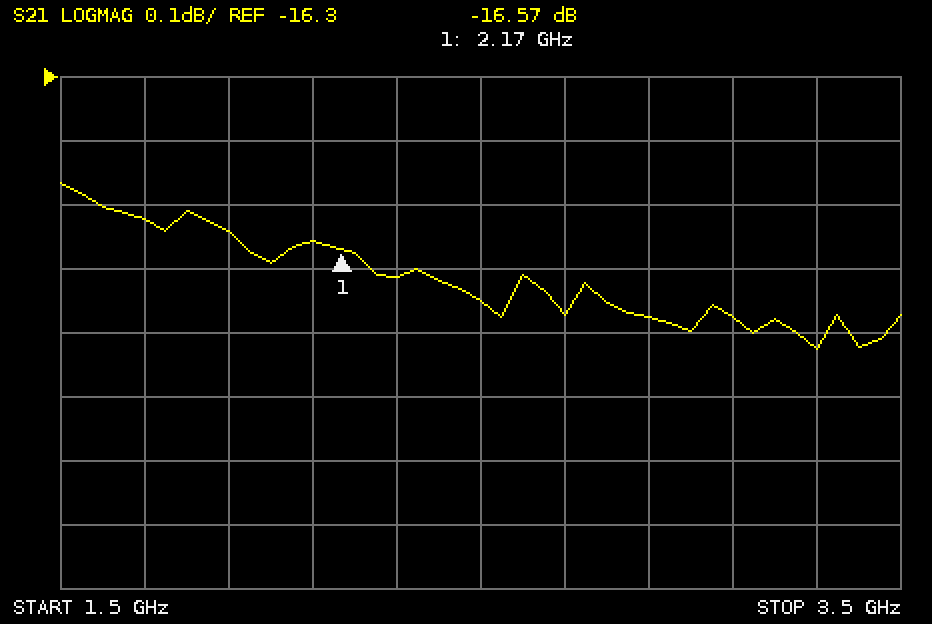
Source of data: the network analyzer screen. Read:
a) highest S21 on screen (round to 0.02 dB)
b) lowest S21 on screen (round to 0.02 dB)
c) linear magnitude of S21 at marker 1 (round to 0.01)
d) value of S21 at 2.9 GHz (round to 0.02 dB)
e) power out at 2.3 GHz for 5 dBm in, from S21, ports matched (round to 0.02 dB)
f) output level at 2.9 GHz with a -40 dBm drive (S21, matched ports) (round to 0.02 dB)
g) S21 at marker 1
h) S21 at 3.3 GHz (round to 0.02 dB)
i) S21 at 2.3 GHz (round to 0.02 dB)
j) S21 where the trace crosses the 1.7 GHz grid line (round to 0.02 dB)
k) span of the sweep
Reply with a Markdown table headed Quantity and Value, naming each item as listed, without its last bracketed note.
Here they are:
| Quantity | Value |
|---|---|
| highest S21 on screen | -16.46 dB |
| lowest S21 on screen | -16.72 dB |
| linear magnitude of S21 at marker 1 | 0.15 |
| value of S21 at 2.9 GHz | -16.68 dB |
| power out at 2.3 GHz for 5 dBm in, from S21, ports matched | -11.62 dBm |
| output level at 2.9 GHz with a -40 dBm drive (S21, matched ports) | -56.68 dBm |
| S21 at marker 1 | -16.57 dB |
| S21 at 3.3 GHz | -16.72 dB |
| S21 at 2.3 GHz | -16.62 dB |
| S21 where the trace crosses the 1.7 GHz grid line | -16.52 dB |
| span of the sweep | 2 GHz |
